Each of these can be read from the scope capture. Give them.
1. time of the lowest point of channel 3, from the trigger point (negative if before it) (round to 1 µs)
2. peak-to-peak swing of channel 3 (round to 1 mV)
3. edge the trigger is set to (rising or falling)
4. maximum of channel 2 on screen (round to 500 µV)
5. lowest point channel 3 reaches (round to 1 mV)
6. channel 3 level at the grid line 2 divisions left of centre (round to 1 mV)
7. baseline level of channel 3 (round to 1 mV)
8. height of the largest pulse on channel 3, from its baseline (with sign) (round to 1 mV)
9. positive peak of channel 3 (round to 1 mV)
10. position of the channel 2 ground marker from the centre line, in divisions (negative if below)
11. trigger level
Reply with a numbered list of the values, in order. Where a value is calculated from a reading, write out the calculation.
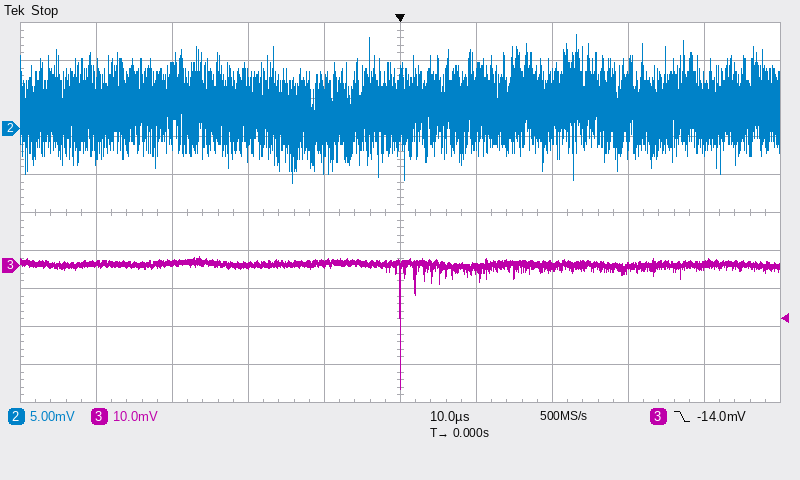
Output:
1. 0 µs
2. 2 mV − (-33 mV) = 35 mV
3. falling
4. 12.5 mV
5. -33 mV
6. 0 mV
7. 0 mV
8. -33 mV − (0 mV) = -33 mV
9. 2 mV
10. +2.2 div
11. -14.0 mV
